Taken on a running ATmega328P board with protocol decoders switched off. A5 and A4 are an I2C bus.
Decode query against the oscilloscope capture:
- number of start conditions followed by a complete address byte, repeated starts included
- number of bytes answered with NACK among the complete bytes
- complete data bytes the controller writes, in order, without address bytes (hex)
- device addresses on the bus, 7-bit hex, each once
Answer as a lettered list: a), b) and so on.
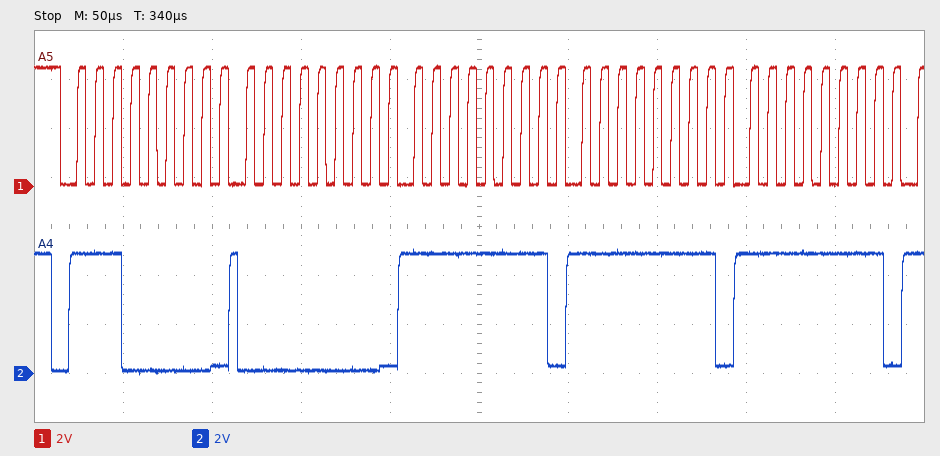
a) 1
b) 0
c) 00 FF FF FF
d) 0x70
